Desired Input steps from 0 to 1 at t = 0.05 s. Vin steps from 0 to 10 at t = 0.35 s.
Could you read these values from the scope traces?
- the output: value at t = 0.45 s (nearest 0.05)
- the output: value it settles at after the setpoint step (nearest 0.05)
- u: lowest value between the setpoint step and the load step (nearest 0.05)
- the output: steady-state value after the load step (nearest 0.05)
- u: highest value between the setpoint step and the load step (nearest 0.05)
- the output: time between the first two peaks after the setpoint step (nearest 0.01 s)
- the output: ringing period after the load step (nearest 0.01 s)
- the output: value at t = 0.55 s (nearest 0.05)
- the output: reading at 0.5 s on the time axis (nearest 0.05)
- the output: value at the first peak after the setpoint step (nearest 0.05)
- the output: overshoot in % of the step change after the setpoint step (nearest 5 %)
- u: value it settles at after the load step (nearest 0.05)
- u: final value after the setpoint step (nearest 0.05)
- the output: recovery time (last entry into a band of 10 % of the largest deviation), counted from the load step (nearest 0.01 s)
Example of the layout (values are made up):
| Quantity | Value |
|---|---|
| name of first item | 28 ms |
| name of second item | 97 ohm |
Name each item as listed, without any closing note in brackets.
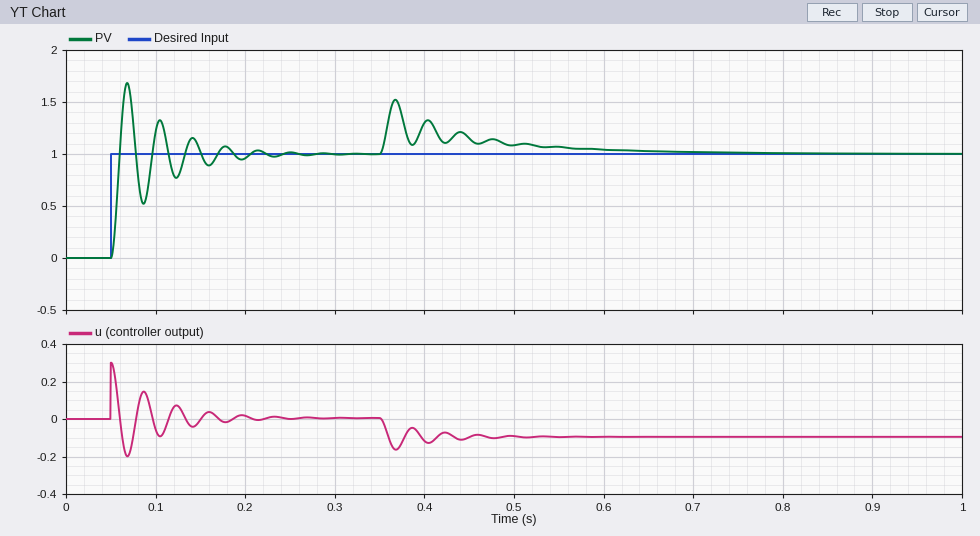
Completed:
| Quantity | Value |
|---|---|
| the output: value at t = 0.45 s | 1.15 |
| the output: value it settles at after the setpoint step | 1.00 |
| u: lowest value between the setpoint step and the load step | -0.20 |
| the output: steady-state value after the load step | 1.00 |
| u: highest value between the setpoint step and the load step | 0.30 |
| the output: time between the first two peaks after the setpoint step | 0.04 s |
| the output: ringing period after the load step | 0.04 s |
| the output: value at t = 0.55 s | 1.05 |
| the output: reading at 0.5 s on the time axis | 1.10 |
| the output: value at the first peak after the setpoint step | 1.70 |
| the output: overshoot in % of the step change after the setpoint step | 70 % |
| u: value it settles at after the load step | -0.10 |
| u: final value after the setpoint step | 0.00 |
| the output: recovery time (last entry into a band of 10 % of the largest deviation), counted from the load step | 0.22 s |
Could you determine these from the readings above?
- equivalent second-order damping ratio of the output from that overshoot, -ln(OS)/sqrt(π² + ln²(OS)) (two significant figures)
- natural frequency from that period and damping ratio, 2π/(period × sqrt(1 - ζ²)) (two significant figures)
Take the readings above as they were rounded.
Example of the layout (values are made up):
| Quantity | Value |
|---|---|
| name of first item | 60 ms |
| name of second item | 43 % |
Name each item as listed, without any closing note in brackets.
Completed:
| Quantity | Value |
|---|---|
| equivalent second-order damping ratio of the output from that overshoot, -ln(OS)/sqrt(π² + ln²(OS)) | 0.11 |
| natural frequency from that period and damping ratio, 2π/(period × sqrt(1 - ζ²)) | 160 rad/s |
